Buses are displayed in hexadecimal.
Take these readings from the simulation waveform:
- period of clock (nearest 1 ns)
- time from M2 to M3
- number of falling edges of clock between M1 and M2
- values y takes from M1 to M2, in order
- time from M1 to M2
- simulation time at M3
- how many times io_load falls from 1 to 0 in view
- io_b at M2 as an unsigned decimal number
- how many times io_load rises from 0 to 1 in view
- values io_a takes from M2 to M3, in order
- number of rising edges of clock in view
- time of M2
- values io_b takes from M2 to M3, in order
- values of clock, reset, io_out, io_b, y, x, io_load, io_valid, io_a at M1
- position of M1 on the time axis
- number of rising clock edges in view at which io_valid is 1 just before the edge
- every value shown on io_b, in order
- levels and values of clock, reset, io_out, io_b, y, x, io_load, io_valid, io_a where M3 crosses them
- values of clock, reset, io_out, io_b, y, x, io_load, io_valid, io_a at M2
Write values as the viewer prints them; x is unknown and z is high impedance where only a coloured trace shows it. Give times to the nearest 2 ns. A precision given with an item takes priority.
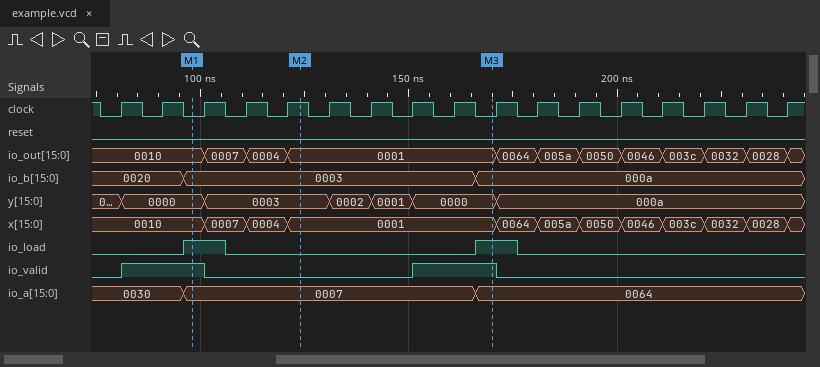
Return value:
10 ns
46 ns
2
0000, 0003
26 ns
170 ns
2
3
2
0007, 0064
17
124 ns
0003, 000a
clock=0, reset=0, io_out=0010, io_b=0003, y=0000, x=0010, io_load=1, io_valid=1, io_a=0007
98 ns
4
0020, 0003, 000a
clock=0, reset=0, io_out=0001, io_b=000a, y=0000, x=0001, io_load=1, io_valid=1, io_a=0064
clock=1, reset=0, io_out=0001, io_b=0003, y=0003, x=0001, io_load=0, io_valid=0, io_a=0007
